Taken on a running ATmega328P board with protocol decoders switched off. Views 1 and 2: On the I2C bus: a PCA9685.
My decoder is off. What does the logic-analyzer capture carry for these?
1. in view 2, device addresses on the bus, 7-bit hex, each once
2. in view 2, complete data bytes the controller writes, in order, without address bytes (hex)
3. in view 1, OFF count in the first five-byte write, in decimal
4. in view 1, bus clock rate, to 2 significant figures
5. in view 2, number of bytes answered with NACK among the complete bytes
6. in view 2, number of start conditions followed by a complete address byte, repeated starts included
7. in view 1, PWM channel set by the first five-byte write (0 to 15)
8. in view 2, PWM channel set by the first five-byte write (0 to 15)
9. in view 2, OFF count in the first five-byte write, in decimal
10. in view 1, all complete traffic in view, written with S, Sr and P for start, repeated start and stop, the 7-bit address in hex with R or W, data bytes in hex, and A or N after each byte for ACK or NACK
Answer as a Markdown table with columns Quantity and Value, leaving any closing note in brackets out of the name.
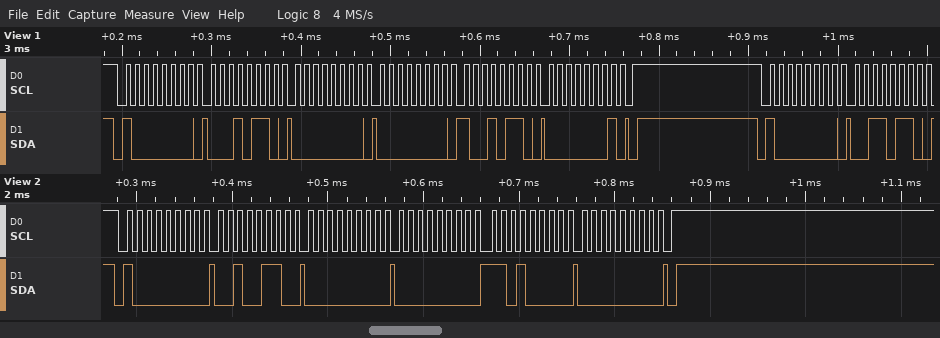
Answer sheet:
| Quantity | Value |
|---|---|
| in view 2, device addresses on the bus, 7-bit hex, each once | 0x40 |
| in view 2, complete data bytes the controller writes, in order, without address bytes | 26 00 00 D0 00 |
| in view 1, OFF count in the first five-byte write, in decimal | 406 |
| in view 1, bus clock rate, to 2 significant figures | 100 kHz |
| in view 2, number of bytes answered with NACK among the complete bytes | 0 |
| in view 2, number of start conditions followed by a complete address byte, repeated starts included | 1 |
| in view 1, PWM channel set by the first five-byte write | 4 |
| in view 2, PWM channel set by the first five-byte write | 8 |
| in view 2, OFF count in the first five-byte write, in decimal | 208 |
| in view 1, all complete traffic in view, written with S, Sr and P for start, repeated start and stop, the 7-bit address in hex with R or W, data bytes in hex, and A or N after each byte for ACK or NACK | S 40W A 16 A 00 A 00 A 96 A 01 A P S 40W A 36 A |
